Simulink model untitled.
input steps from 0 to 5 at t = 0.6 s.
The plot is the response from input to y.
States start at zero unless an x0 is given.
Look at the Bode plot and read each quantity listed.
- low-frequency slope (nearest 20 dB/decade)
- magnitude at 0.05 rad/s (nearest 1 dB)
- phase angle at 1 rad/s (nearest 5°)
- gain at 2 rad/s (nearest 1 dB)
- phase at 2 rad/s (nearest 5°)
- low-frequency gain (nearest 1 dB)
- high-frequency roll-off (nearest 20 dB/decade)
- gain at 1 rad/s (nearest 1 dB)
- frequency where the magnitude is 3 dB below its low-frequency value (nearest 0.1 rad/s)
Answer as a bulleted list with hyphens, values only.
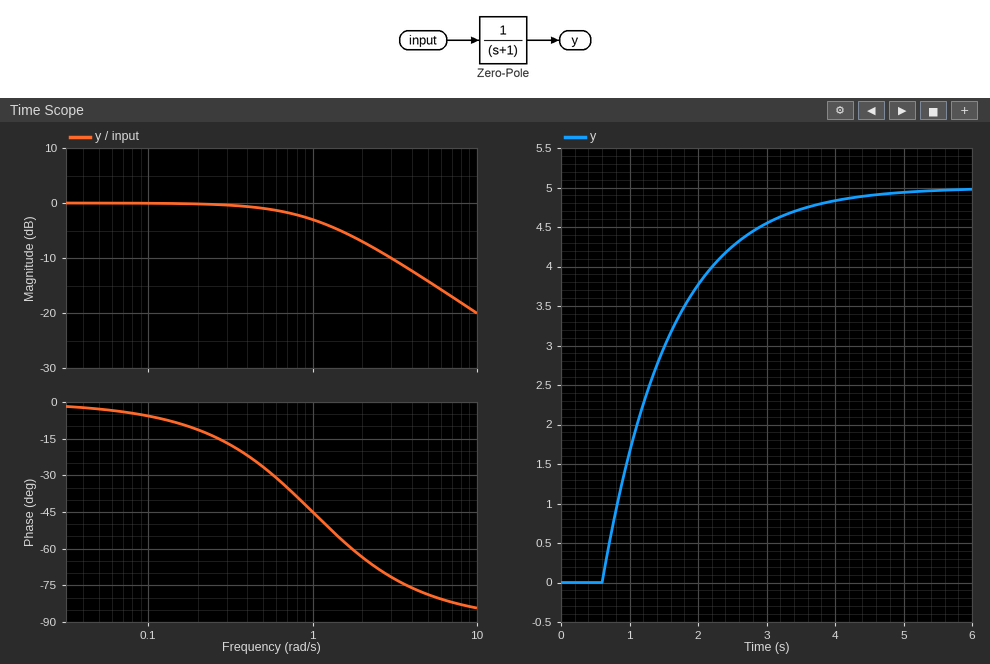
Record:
- 0 dB/decade
- 0 dB
- -45°
- -7 dB
- -65°
- 0 dB
- -20 dB/decade
- -3 dB
- 1.0 rad/s
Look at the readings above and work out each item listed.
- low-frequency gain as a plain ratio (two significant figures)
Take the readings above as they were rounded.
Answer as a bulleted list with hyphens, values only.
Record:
- 1.0
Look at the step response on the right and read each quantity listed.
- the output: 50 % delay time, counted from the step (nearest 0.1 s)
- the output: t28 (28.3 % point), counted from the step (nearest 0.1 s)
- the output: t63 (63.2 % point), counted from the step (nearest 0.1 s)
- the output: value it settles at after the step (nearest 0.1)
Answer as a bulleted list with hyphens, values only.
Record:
- 0.7 s
- 0.3 s
- 1.0 s
- 5.0
